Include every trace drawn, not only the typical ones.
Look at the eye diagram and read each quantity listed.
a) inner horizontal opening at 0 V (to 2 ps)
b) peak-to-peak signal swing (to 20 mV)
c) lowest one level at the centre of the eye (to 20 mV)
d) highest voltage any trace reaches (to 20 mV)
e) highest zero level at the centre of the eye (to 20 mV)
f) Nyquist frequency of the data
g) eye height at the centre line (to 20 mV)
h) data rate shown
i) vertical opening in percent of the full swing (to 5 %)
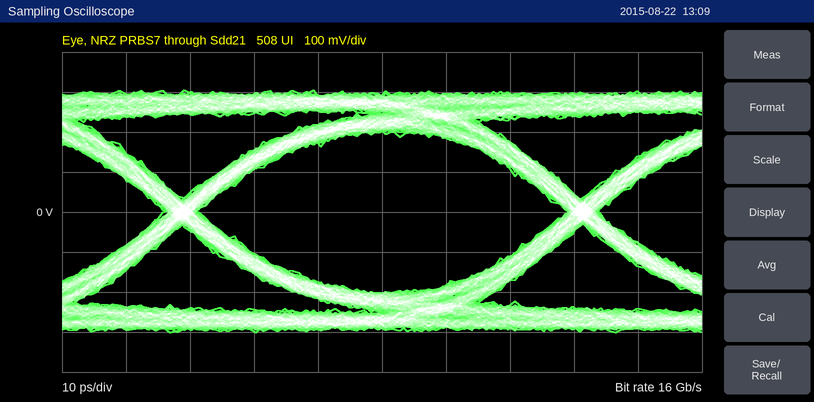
58 ps
600 mV
200 mV
300 mV
-200 mV
8 GHz
400 mV
16 Gb/s
65 %
